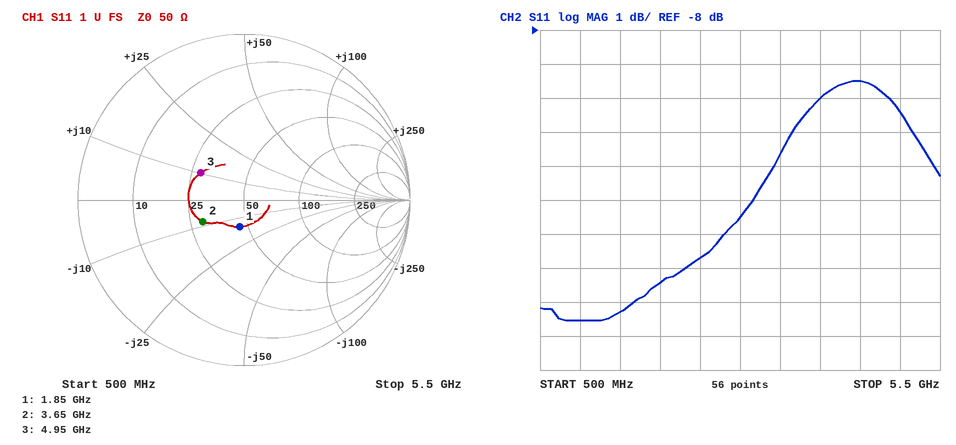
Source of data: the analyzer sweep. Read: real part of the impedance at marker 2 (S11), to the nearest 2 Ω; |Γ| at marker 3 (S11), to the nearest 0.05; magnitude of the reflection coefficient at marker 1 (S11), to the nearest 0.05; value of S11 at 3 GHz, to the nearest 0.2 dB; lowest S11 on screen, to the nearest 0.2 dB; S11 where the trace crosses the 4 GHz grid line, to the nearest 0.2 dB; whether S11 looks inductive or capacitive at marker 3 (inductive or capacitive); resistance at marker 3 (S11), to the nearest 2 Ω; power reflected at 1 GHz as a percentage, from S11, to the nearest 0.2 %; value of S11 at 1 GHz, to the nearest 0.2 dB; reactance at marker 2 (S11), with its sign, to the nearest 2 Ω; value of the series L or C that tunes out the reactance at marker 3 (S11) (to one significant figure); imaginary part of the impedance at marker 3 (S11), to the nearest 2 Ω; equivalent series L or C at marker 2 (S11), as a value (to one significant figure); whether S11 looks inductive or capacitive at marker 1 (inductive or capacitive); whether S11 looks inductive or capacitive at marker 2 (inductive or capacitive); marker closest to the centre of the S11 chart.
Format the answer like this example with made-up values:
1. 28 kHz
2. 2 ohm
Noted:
1. 30 Ω
2. 0.30
3. 0.15
4. -13.6 dB
5. -16.6 dB
6. -10.0 dB
7. inductive
8. 28 Ω
9. 2.2 %
10. -16.6 dB
11. -8 Ω
12. 3 pF
13. +10 Ω
14. 5 pF
15. capacitive
16. capacitive
17. marker 1
